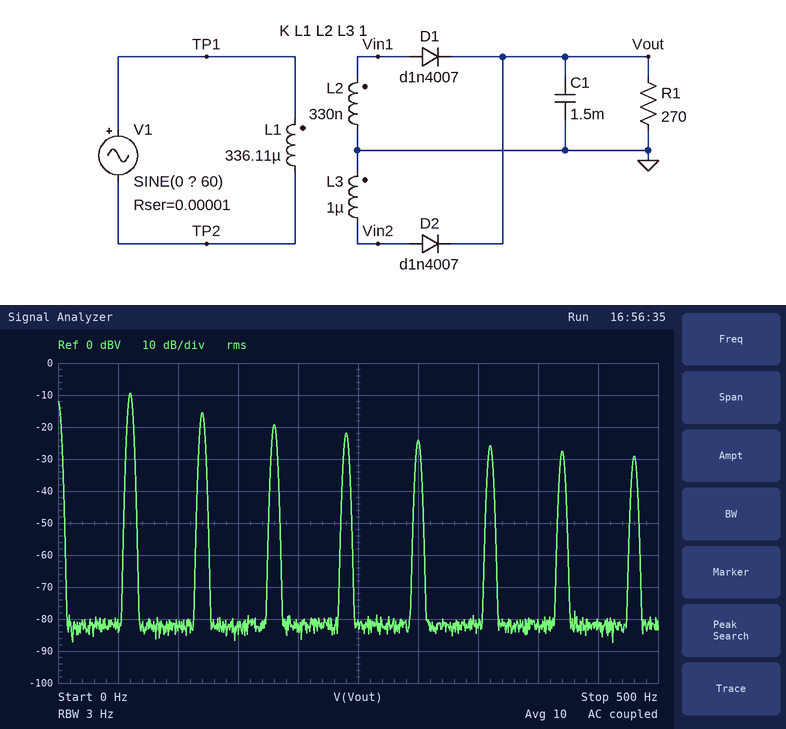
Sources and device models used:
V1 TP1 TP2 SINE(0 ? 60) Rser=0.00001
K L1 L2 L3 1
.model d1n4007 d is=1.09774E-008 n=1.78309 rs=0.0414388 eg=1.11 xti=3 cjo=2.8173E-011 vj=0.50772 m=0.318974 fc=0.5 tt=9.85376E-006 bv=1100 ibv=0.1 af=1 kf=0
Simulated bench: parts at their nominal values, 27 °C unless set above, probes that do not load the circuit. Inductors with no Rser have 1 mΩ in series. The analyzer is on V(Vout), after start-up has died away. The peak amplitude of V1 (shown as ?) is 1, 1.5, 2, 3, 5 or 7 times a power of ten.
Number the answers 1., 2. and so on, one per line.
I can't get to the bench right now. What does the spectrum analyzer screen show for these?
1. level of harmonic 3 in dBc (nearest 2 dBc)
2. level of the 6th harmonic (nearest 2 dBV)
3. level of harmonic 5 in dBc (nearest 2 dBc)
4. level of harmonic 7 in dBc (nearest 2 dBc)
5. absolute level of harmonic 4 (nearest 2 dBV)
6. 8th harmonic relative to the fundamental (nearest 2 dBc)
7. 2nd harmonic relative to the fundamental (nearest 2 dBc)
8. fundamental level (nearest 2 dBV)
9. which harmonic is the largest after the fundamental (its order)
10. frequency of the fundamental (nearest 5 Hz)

1. -10 dBc
2. -26 dBV
3. -14 dBc
4. -18 dBc
5. -22 dBV
6. -20 dBc
7. -6 dBc
8. -10 dBV
9. 2
10. 60 Hz
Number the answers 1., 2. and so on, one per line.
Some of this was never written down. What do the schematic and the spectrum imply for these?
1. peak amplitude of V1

1. 700 V
